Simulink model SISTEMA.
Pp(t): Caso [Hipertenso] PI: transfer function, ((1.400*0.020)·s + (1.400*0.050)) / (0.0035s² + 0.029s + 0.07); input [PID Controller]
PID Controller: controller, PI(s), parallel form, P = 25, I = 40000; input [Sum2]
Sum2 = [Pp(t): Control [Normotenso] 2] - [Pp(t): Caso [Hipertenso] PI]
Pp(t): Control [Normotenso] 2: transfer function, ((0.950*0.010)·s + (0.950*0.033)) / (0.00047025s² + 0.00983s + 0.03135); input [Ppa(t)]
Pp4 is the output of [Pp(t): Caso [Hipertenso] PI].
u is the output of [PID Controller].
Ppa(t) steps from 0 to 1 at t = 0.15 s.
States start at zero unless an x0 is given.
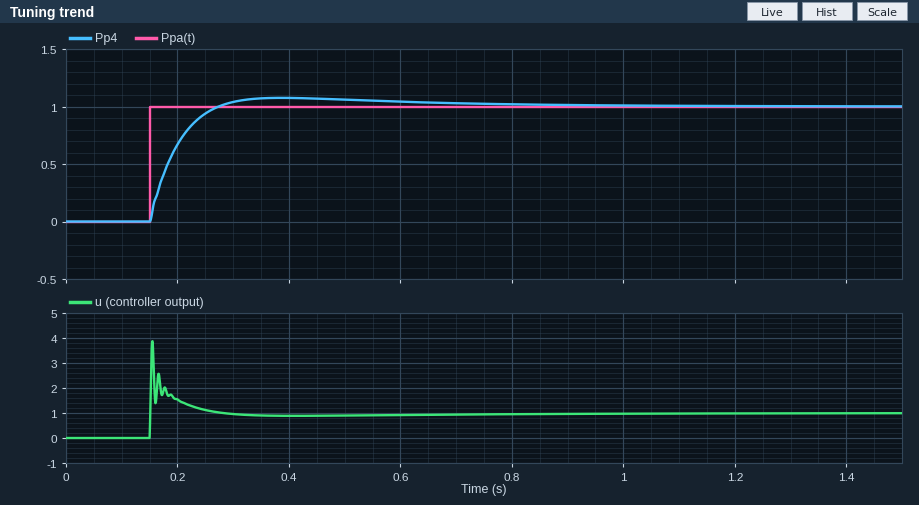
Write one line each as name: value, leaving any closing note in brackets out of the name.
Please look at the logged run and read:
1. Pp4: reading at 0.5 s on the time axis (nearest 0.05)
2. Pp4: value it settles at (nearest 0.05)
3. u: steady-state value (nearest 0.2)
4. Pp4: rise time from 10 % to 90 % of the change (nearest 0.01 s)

Pp4: reading at 0.5 s on the time axis: 1.05
Pp4: value it settles at: 1.00
u: steady-state value: 1.0
Pp4: rise time from 10 % to 90 % of the change: 0.08 s
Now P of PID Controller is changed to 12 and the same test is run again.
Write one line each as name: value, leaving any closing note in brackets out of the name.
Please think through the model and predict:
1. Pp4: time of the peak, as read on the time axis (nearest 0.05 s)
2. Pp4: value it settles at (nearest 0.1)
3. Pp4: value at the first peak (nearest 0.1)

Pp4: time of the peak, as read on the time axis: 0.40 s
Pp4: value it settles at: 1.0
Pp4: value at the first peak: 1.1
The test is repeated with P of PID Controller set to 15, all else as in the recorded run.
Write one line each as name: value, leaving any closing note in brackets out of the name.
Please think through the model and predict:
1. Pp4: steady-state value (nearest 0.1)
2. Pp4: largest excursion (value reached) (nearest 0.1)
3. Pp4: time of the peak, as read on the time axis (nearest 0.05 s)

Pp4: steady-state value: 1.0
Pp4: largest excursion (value reached): 1.1
Pp4: time of the peak, as read on the time axis: 0.40 s
